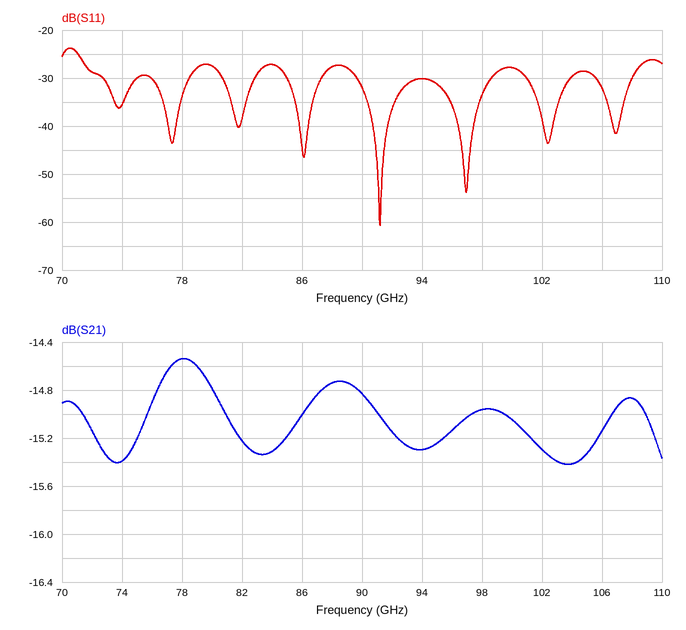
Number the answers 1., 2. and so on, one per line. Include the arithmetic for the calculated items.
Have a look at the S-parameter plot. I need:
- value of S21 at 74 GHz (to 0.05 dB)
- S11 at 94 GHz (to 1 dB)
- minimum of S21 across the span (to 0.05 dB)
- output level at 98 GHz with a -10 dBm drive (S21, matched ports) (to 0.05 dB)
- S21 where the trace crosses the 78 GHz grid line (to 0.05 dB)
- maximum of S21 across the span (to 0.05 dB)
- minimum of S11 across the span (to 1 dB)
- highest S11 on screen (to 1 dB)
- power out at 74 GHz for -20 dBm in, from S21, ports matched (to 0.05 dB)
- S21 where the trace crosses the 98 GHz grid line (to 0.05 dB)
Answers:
1. -15.40 dB
2. -30 dB
3. -15.40 dB
4. -10 dBm + (-14.95 dB) = -24.95 dBm
5. -14.55 dB
6. -14.55 dB
7. -61 dB
8. -24 dB
9. -20 dBm + (-15.40 dB) = -35.40 dBm
10. -14.95 dB
